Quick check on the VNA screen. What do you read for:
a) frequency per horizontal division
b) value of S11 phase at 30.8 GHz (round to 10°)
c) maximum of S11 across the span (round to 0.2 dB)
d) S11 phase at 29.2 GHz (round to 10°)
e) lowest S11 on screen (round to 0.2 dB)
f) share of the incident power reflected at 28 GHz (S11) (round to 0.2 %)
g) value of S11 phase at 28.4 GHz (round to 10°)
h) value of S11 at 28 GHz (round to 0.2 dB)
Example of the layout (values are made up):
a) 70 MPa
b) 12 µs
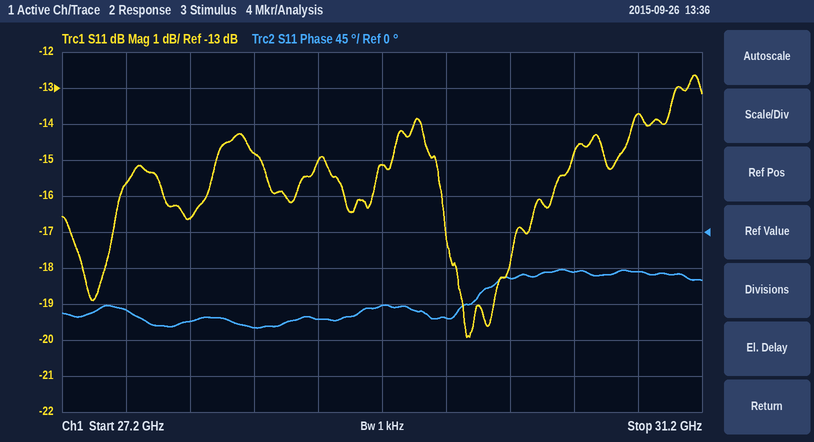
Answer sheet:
a) 400 MHz
b) -50°
c) -12.6 dB
d) -90°
e) -20.0 dB
f) 2.2 %
g) -120°
h) -16.6 dB
